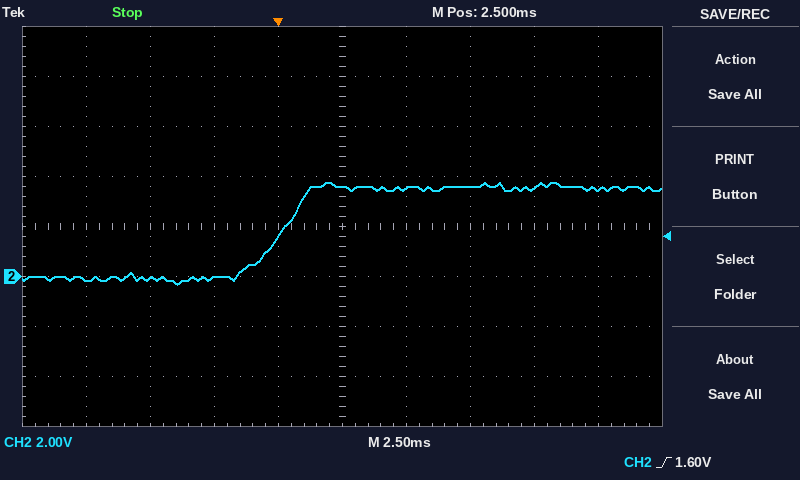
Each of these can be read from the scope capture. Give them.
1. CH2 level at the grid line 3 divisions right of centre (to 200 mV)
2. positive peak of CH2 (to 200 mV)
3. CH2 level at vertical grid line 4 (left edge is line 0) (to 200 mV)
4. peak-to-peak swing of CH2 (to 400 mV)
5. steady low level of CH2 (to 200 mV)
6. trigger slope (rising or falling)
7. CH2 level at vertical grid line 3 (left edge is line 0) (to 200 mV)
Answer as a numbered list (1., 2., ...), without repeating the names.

1. 3.6 V
2. 3.8 V
3. 1.6 V
4. 4.0 V
5. 0.0 V
6. rising
7. 0.0 V
